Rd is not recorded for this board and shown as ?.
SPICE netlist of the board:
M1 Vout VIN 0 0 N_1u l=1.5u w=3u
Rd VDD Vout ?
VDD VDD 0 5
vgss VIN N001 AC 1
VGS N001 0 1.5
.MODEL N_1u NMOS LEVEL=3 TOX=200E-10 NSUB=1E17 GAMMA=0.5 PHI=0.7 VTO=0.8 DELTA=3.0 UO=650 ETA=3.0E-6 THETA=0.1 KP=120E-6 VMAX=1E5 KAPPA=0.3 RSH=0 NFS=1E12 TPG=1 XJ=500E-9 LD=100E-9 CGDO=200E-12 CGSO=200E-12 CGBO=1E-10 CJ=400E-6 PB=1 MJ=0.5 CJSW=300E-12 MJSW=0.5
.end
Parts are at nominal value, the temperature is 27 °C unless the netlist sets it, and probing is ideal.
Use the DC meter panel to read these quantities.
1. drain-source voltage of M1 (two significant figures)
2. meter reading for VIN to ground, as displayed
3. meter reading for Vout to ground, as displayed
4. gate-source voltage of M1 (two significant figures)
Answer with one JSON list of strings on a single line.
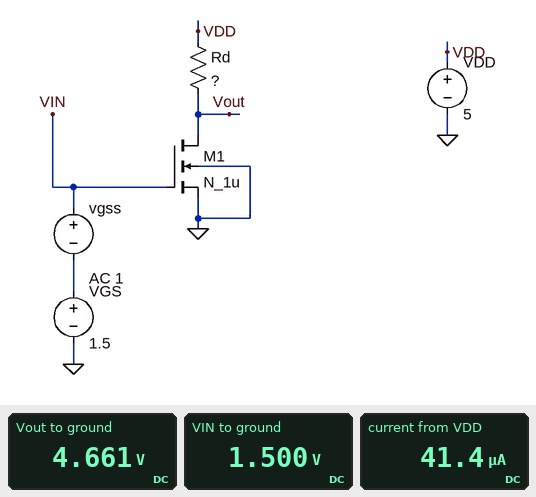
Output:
["4.7 V", "1.500 V", "4.661 V", "1.5 V"]
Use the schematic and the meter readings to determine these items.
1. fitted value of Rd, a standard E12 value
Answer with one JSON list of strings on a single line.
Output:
["8.2 kΩ"]
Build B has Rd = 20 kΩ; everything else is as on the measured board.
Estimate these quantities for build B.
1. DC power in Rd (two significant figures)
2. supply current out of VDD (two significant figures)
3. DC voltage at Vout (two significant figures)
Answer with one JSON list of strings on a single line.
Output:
["34 µW", "41 µA", "4.2 V"]
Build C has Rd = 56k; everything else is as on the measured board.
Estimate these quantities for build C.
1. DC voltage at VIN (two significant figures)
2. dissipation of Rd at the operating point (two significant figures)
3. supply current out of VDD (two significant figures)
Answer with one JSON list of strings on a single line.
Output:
["1.5 V", "91 µW", "40 µA"]
